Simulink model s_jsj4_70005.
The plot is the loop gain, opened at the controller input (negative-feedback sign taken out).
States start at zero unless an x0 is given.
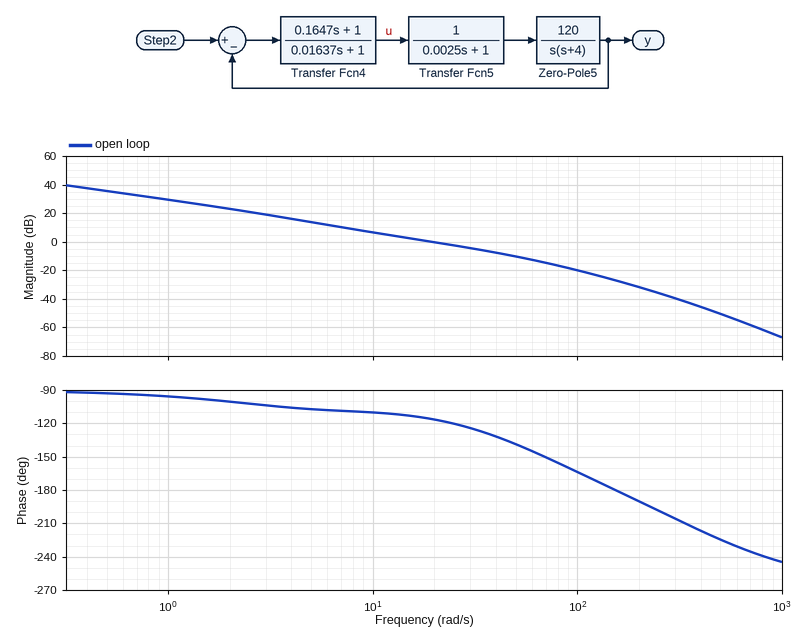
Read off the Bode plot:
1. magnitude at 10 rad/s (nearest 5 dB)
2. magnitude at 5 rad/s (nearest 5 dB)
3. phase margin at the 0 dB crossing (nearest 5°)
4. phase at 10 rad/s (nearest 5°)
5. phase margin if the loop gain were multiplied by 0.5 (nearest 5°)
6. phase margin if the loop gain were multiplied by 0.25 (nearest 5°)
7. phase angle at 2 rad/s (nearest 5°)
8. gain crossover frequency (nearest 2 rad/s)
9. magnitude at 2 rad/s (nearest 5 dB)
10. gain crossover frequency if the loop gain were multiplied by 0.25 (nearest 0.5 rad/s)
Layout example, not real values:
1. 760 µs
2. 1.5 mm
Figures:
1. 5 dB
2. 15 dB
3. 65°
4. -110°
5. 70°
6. 70°
7. -100°
8. 20 rad/s
9. 25 dB
10. 6.0 rad/s
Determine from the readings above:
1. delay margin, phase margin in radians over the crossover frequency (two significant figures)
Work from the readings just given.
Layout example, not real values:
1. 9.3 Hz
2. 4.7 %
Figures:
1. 0.057 s
